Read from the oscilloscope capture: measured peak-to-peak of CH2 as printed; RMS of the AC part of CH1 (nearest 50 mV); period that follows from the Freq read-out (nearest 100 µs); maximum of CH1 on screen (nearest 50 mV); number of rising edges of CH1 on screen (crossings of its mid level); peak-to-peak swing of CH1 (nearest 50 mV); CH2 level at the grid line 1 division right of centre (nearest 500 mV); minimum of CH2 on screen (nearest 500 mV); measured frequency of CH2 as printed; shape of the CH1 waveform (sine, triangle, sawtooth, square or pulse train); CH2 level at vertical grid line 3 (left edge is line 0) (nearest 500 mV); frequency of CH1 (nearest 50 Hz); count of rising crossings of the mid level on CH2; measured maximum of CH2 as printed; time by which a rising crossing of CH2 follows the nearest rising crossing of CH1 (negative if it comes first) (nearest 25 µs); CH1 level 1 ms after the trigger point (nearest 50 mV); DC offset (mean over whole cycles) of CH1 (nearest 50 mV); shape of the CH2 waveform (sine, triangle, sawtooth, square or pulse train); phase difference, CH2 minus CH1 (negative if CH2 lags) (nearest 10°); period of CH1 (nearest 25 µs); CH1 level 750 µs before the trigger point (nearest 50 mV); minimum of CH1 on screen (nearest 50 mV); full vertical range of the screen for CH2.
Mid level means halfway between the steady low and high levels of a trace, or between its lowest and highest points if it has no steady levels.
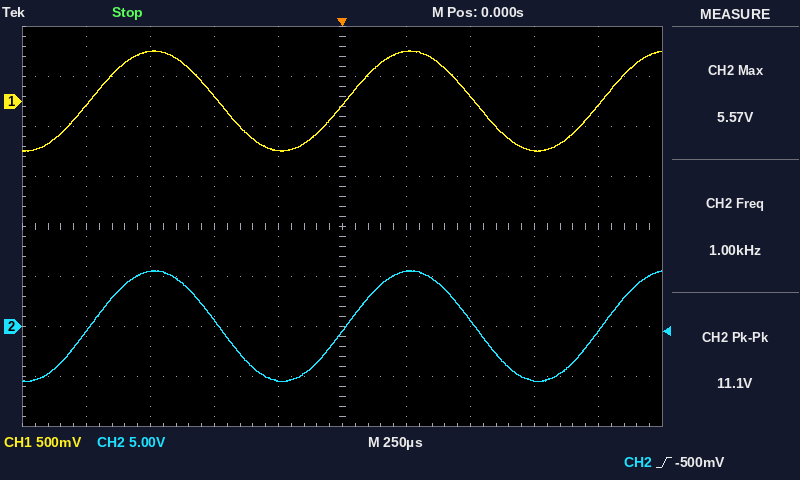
11.1 V
350 mV
1.0 ms
500 mV
3
1.00 V
5.5 V
-5.5 V
1.00 kHz
sine
500 mV
1.00 kHz
3
5.57 V
0 µs
-50 mV
0 mV
sine
0°
1.000 ms
500 mV
-500 mV
40 V
